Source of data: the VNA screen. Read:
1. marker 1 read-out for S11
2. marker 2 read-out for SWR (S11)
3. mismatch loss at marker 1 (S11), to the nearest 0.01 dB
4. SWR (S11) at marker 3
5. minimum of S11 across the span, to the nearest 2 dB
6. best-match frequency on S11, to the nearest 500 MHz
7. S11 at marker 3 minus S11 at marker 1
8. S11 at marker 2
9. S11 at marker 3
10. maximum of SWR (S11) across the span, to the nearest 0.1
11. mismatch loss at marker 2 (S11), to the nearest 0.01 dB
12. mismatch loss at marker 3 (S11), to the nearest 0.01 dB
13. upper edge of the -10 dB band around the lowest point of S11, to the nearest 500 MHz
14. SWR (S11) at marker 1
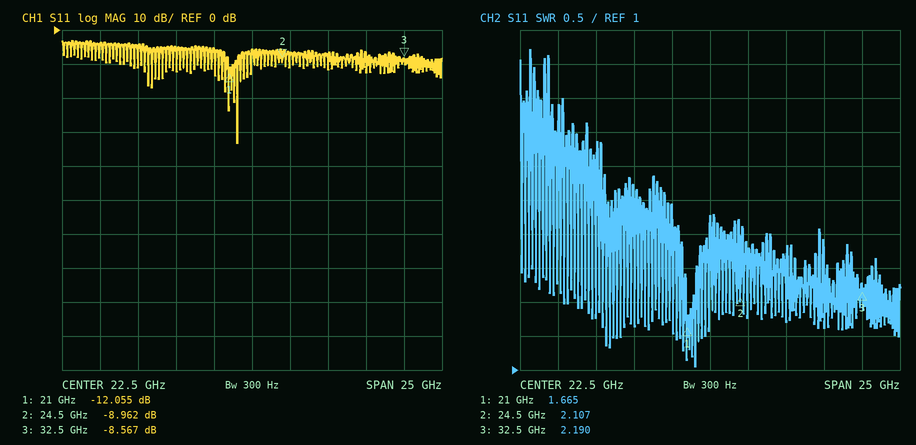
-12.055 dB
2.107
0.28 dB
2.190
-34 dB
21.5 GHz
3.488 dB
-8.962 dB
-8.567 dB
5.7
0.59 dB
0.65 dB
21.5 GHz
1.665
